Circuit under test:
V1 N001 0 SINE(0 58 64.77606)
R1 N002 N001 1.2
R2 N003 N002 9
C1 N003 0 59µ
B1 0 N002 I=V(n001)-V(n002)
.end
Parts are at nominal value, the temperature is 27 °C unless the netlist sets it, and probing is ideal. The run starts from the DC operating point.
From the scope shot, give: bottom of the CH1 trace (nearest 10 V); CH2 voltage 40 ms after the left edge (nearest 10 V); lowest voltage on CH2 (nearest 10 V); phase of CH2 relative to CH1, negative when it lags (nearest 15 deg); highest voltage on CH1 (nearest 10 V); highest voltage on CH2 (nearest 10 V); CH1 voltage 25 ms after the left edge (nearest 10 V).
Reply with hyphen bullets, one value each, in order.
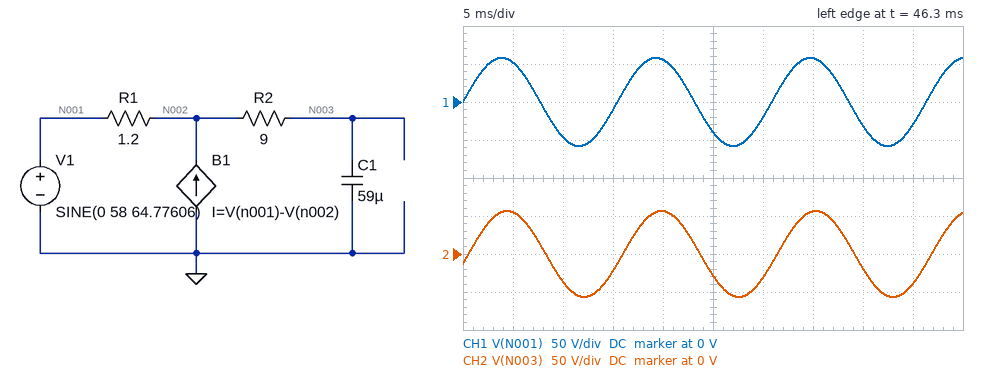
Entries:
- -60 V
- -20 V
- -60 V
- -15 deg
- 60 V
- 60 V
- -40 V
